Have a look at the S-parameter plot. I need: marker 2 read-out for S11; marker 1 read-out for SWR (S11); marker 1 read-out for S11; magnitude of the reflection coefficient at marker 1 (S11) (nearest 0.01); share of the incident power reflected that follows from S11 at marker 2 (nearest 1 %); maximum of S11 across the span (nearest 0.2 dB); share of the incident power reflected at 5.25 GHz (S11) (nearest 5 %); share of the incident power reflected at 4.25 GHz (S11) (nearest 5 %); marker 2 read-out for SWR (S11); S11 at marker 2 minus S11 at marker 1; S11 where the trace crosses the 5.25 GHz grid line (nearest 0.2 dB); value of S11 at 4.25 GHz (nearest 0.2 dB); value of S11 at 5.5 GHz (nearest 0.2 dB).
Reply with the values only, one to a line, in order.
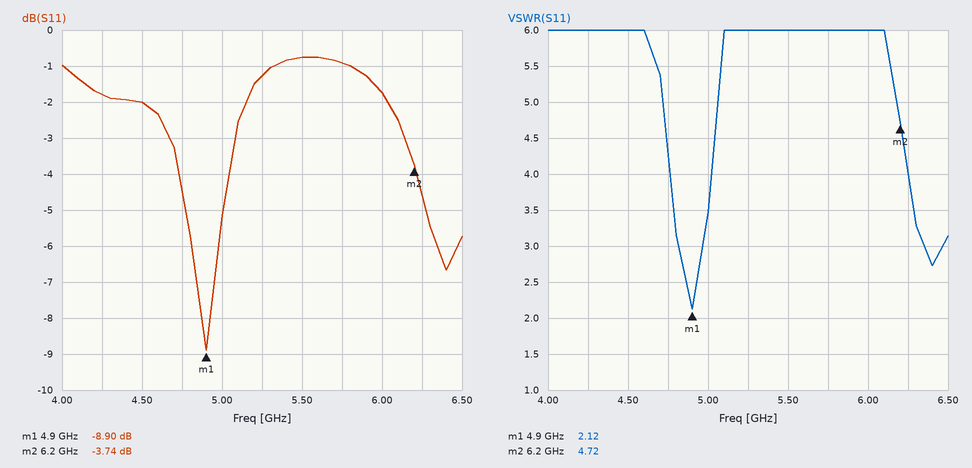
-3.74 dB
2.12
-8.90 dB
0.36
42 %
-0.8 dB
75 %
65 %
4.72
5.16 dB
-1.2 dB
-1.8 dB
-0.8 dB
